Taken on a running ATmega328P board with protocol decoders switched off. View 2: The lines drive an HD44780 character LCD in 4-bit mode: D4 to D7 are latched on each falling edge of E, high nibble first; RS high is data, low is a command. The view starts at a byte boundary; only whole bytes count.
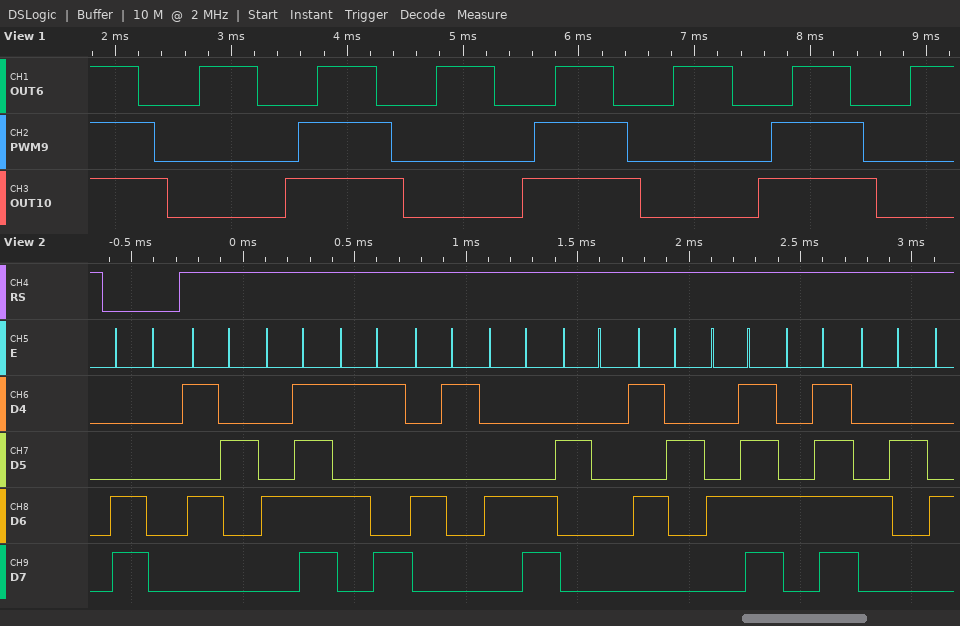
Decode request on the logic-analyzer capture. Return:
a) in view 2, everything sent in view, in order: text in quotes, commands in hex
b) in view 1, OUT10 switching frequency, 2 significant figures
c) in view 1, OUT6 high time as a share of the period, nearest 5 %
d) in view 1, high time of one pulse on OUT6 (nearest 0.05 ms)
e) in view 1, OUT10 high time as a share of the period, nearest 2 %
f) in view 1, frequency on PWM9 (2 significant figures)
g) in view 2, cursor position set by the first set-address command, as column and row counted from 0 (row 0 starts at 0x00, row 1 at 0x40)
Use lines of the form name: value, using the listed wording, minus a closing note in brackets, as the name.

in view 2, everything sent in view, in order: text in quotes, commands in hex: 0xC0 "ROYAL ROOB"
in view 1, OUT10 switching frequency, 2 significant figures: 490 Hz
in view 1, OUT6 high time as a share of the period, nearest 5 %: 50 %
in view 1, high time of one pulse on OUT6: 0.50 ms
in view 1, OUT10 high time as a share of the period, nearest 2 %: 50 %
in view 1, frequency on PWM9: 490 Hz
in view 2, cursor position set by the first set-address command, as column and row counted from 0: column 0, row 1
